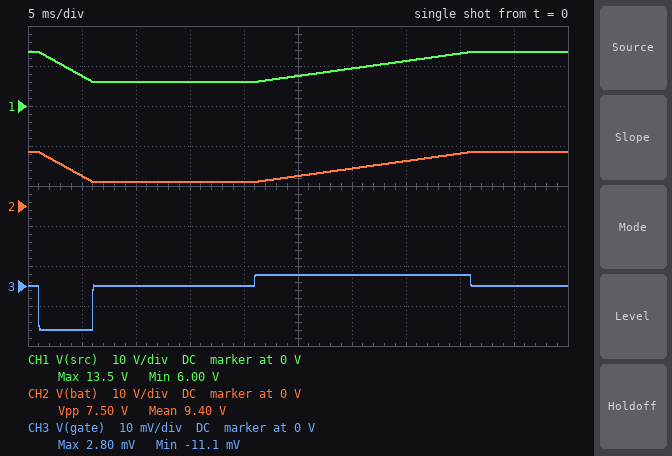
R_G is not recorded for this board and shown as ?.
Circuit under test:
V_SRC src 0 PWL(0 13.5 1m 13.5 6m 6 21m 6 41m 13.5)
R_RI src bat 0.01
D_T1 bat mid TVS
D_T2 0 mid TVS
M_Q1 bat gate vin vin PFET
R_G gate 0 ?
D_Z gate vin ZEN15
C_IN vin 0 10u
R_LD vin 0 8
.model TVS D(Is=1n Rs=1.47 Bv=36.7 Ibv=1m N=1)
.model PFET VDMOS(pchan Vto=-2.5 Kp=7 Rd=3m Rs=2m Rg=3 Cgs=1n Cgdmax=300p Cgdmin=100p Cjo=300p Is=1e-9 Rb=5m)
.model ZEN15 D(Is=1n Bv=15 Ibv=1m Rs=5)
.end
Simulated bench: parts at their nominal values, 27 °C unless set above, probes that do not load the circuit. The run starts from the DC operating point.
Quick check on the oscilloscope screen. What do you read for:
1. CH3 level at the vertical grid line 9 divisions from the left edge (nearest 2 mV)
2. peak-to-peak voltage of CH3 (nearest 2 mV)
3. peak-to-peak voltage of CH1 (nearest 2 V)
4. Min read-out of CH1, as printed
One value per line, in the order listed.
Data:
0 V
14 mV
8 V
6.00 V
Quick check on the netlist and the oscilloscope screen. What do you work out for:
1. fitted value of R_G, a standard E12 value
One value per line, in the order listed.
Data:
5.6 kΩ
